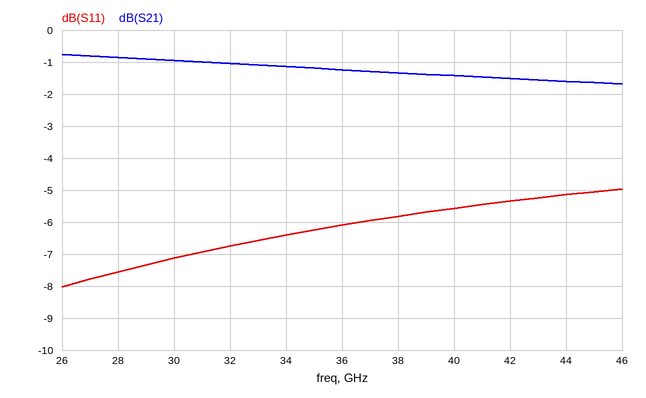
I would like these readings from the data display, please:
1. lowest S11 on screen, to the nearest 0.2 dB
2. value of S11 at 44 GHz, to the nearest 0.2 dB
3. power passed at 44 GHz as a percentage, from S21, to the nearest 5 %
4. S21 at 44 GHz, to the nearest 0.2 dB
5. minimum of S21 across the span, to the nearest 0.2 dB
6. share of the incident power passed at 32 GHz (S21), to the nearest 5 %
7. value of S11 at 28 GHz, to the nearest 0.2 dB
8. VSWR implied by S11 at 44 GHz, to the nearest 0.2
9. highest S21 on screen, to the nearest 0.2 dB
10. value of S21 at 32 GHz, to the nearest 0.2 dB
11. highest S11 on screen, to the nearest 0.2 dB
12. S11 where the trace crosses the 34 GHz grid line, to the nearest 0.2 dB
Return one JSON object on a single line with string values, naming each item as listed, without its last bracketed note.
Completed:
{"lowest S11 on screen, to the nearest 0.2 dB": "-8.0 dB", "value of S11 at 44 GHz, to the nearest 0.2 dB": "-5.2 dB", "power passed at 44 GHz as a percentage, from S21, to the nearest 5 %": "70 %", "S21 at 44 GHz, to the nearest 0.2 dB": "-1.6 dB", "minimum of S21 across the span, to the nearest 0.2 dB": "-1.6 dB", "share of the incident power passed at 32 GHz (S21), to the nearest 5 %": "80 %", "value of S11 at 28 GHz, to the nearest 0.2 dB": "-7.6 dB", "VSWR implied by S11 at 44 GHz, to the nearest 0.2": "3.4", "highest S21 on screen, to the nearest 0.2 dB": "-0.8 dB", "value of S21 at 32 GHz, to the nearest 0.2 dB": "-1.0 dB", "highest S11 on screen, to the nearest 0.2 dB": "-5.0 dB", "S11 where the trace crosses the 34 GHz grid line, to the nearest 0.2 dB": "-6.4 dB"}
